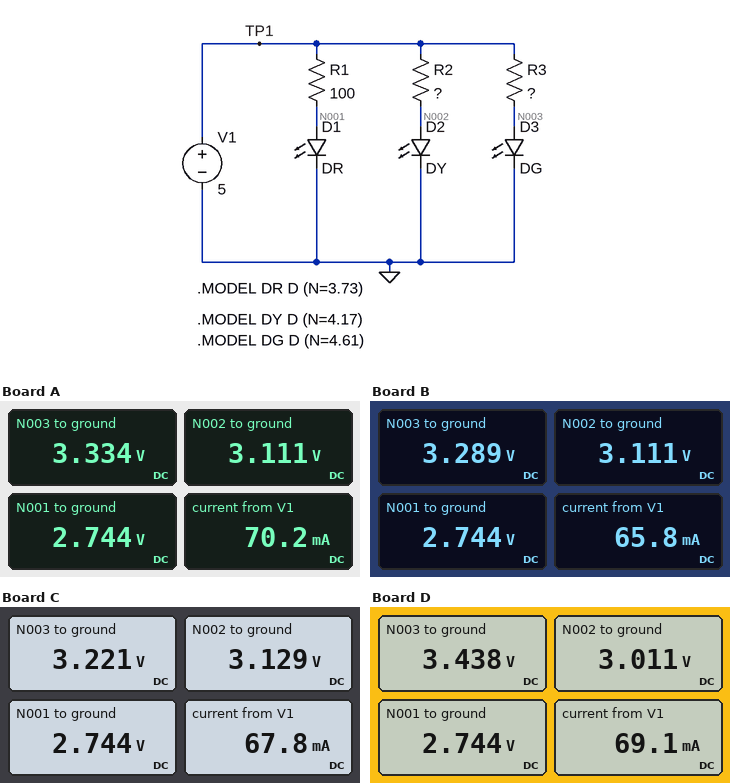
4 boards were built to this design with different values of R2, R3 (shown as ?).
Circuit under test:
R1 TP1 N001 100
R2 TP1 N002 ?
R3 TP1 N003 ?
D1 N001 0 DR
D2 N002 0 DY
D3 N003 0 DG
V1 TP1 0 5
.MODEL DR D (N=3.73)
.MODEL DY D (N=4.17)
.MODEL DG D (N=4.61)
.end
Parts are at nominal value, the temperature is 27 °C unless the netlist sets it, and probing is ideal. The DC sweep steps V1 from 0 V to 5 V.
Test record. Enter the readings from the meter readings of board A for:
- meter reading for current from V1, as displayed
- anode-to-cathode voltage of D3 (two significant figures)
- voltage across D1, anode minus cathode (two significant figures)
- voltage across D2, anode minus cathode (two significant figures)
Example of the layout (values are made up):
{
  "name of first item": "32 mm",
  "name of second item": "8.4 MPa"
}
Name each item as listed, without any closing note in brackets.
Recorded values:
{
  "meter reading for current from V1, as displayed": "70.2 mA",
  "anode-to-cathode voltage of D3": "3.3 V",
  "voltage across D1, anode minus cathode": "2.7 V",
  "voltage across D2, anode minus cathode": "3.1 V"
}
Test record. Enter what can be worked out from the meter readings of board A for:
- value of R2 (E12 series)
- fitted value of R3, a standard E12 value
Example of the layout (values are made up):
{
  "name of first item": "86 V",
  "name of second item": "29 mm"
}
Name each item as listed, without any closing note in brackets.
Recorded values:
{
  "value of R2": "56 Ω",
  "fitted value of R3, a standard E12 value": "120 Ω"
}
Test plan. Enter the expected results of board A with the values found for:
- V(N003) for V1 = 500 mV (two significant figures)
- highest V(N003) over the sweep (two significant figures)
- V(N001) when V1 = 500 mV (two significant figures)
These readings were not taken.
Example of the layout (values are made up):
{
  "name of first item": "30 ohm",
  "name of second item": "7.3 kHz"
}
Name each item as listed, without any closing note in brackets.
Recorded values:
{
  "V(N003) for V1 = 500 mV": "500 mV",
  "highest V(N003) over the sweep": "3.3 V",
  "V(N001) when V1 = 500 mV": "500 mV"
}
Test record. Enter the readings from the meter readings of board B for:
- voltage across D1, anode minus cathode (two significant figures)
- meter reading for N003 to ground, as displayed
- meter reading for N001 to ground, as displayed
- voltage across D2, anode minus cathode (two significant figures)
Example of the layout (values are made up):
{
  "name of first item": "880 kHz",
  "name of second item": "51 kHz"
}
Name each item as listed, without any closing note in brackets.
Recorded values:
{
  "voltage across D1, anode minus cathode": "2.7 V",
  "meter reading for N003 to ground, as displayed": "3.289 V",
  "meter reading for N001 to ground, as displayed": "2.744 V",
  "voltage across D2, anode minus cathode": "3.1 V"
}
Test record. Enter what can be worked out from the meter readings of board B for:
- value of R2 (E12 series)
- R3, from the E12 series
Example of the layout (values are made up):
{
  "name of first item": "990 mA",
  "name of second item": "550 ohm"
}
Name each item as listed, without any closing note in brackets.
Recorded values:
{
  "value of R2": "56 Ω",
  "R3, from the E12 series": "180 Ω"
}
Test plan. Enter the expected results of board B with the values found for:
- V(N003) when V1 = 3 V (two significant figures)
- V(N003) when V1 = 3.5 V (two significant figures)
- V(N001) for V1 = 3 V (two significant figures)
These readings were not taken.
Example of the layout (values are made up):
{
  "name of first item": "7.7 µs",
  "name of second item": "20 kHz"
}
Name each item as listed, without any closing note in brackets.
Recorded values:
{
  "V(N003) when V1 = 3 V": "2.9 V",
  "V(N003) when V1 = 3.5 V": "3.1 V",
  "V(N001) for V1 = 3 V": "2.6 V"
}
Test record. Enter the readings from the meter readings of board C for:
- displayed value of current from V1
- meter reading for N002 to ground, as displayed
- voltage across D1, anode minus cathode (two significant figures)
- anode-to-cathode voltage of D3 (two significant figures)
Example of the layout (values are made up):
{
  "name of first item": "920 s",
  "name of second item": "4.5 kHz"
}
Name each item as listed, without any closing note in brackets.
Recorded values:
{
  "displayed value of current from V1": "67.8 mA",
  "meter reading for N002 to ground, as displayed": "3.129 V",
  "voltage across D1, anode minus cathode": "2.7 V",
  "anode-to-cathode voltage of D3": "3.2 V"
}
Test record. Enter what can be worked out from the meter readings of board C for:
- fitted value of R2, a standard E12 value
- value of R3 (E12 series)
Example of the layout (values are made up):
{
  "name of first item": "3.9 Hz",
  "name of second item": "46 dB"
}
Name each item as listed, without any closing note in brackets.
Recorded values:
{
  "fitted value of R2, a standard E12 value": "47 Ω",
  "value of R3": "330 Ω"
}
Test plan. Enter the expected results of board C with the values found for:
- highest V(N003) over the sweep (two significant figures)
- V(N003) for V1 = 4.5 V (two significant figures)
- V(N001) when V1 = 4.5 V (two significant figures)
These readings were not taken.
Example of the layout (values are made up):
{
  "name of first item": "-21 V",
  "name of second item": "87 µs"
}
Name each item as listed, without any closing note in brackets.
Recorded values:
{
  "highest V(N003) over the sweep": "3.2 V",
  "V(N003) for V1 = 4.5 V": "3.2 V",
  "V(N001) when V1 = 4.5 V": "2.7 V"
}
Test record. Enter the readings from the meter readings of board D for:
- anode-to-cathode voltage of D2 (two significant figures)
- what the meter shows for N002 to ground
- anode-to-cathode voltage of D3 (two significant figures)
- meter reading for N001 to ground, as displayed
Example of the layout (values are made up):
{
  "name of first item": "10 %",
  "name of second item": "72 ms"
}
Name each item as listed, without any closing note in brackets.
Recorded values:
{
  "anode-to-cathode voltage of D2": "3.0 V",
  "what the meter shows for N002 to ground": "3.011 V",
  "anode-to-cathode voltage of D3": "3.4 V",
  "meter reading for N001 to ground, as displayed": "2.744 V"
}
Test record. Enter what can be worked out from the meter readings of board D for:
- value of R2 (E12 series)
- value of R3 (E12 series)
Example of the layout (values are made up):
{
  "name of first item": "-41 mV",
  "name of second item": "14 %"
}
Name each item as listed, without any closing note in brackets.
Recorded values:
{
  "value of R2": "150 Ω",
  "value of R3": "47 Ω"
}
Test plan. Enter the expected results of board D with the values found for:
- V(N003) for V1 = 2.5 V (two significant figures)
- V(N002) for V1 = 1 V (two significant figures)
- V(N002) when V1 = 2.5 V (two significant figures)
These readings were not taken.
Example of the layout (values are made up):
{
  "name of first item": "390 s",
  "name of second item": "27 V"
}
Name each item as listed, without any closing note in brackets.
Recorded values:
{
  "V(N003) for V1 = 2.5 V": "2.5 V",
  "V(N002) for V1 = 1 V": "1.0 V",
  "V(N002) when V1 = 2.5 V": "2.5 V"
}
